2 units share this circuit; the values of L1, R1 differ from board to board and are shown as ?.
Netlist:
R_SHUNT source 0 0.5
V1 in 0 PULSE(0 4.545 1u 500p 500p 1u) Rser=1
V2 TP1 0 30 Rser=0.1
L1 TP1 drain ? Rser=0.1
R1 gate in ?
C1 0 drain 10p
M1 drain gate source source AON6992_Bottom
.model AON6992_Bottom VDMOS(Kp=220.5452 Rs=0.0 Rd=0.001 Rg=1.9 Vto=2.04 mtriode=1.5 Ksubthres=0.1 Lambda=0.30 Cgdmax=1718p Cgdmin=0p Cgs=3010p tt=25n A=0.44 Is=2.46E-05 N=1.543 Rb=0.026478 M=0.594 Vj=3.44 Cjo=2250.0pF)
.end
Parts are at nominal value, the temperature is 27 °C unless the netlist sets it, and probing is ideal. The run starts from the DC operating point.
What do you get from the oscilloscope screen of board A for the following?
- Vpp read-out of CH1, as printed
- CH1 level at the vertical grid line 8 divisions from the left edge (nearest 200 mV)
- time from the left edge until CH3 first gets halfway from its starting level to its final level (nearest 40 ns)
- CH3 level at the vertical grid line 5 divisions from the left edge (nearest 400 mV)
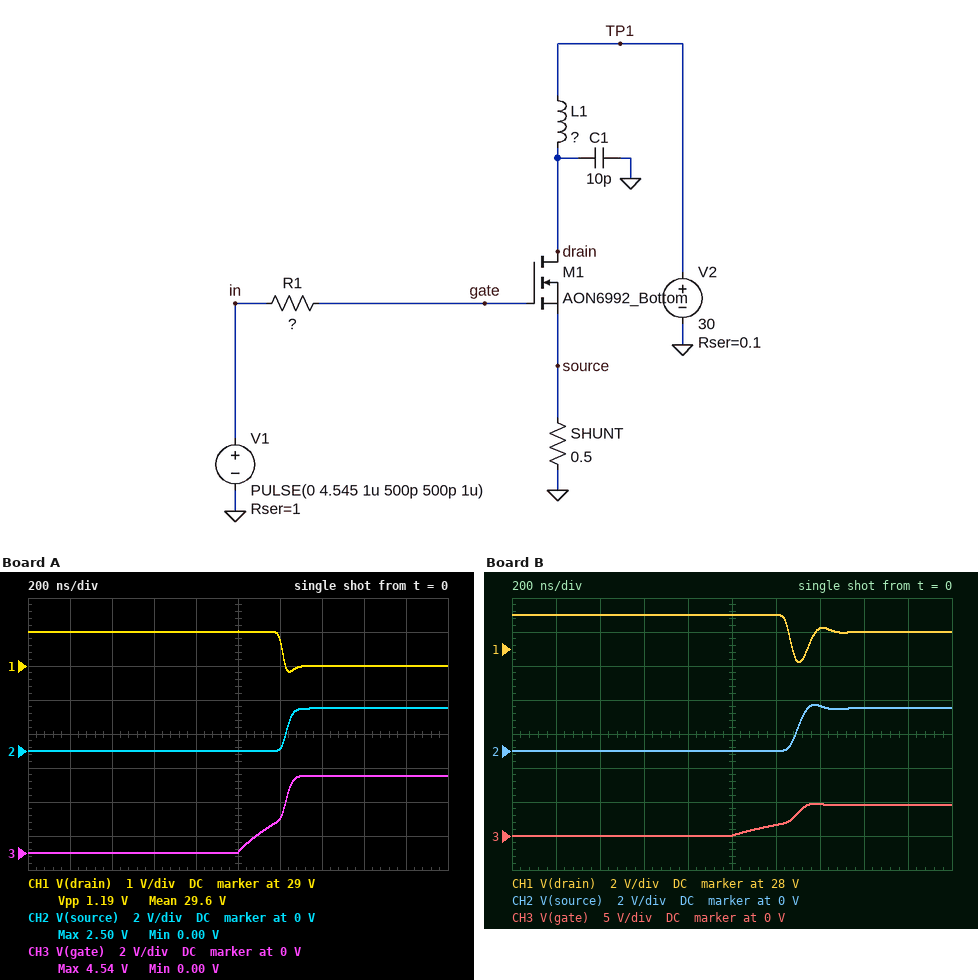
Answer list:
1.19 V
29.0 V
1.20 µs
0 V
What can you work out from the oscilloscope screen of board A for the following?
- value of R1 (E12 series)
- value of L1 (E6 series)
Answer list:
120 Ω
6.8 nH
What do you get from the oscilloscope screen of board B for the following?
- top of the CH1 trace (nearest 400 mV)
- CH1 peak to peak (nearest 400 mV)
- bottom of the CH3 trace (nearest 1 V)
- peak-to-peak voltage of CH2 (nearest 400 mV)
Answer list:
30.0 V
2.8 V
0 V
2.8 V
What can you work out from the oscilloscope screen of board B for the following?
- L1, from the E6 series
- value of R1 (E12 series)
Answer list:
33 nH
150 Ω
